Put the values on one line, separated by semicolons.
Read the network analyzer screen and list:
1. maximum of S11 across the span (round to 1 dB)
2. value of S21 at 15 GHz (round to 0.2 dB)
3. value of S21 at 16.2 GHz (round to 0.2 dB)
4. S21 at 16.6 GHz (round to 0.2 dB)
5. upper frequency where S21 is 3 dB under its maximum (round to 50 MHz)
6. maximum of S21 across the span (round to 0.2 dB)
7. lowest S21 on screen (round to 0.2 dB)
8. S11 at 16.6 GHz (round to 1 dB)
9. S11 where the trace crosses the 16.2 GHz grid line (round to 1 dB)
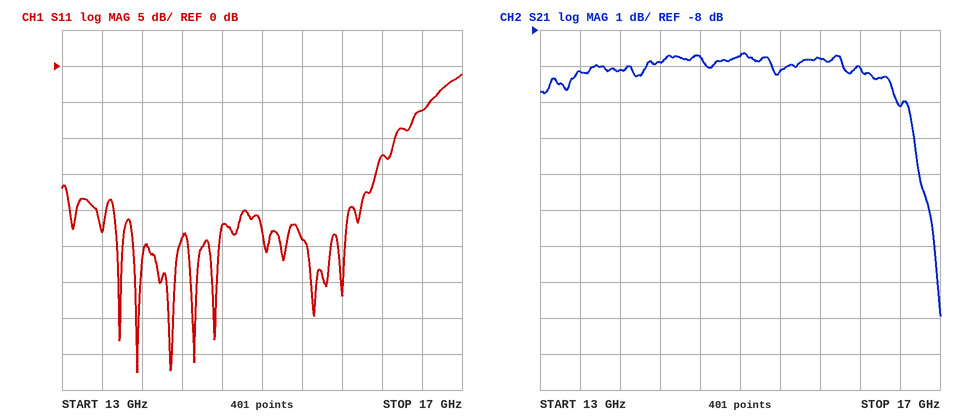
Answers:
-1 dB; -8.8 dB; -9.0 dB; -10.2 dB; 16.75 GHz; -8.6 dB; -16.0 dB; -6 dB; -12 dB
